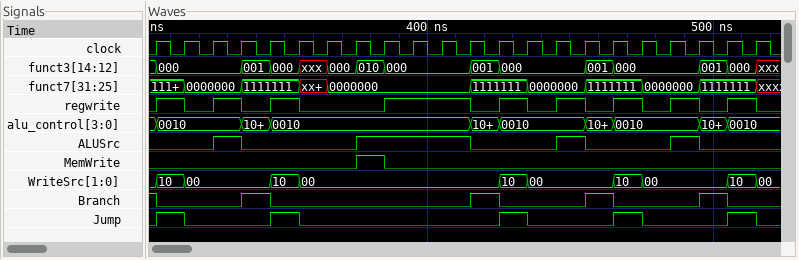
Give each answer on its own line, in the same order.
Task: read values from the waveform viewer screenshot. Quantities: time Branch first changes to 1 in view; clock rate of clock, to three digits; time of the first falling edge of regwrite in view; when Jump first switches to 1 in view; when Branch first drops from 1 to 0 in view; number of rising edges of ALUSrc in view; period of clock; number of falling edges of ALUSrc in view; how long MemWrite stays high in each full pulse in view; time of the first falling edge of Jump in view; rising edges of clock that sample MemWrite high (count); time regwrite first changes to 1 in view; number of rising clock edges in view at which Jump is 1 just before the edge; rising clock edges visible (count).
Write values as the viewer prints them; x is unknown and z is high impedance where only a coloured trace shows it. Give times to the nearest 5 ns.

335 ns
100 MHz
315 ns
305 ns
305 ns
4
10 ns
4
10 ns
315 ns
1
305 ns
5
22
